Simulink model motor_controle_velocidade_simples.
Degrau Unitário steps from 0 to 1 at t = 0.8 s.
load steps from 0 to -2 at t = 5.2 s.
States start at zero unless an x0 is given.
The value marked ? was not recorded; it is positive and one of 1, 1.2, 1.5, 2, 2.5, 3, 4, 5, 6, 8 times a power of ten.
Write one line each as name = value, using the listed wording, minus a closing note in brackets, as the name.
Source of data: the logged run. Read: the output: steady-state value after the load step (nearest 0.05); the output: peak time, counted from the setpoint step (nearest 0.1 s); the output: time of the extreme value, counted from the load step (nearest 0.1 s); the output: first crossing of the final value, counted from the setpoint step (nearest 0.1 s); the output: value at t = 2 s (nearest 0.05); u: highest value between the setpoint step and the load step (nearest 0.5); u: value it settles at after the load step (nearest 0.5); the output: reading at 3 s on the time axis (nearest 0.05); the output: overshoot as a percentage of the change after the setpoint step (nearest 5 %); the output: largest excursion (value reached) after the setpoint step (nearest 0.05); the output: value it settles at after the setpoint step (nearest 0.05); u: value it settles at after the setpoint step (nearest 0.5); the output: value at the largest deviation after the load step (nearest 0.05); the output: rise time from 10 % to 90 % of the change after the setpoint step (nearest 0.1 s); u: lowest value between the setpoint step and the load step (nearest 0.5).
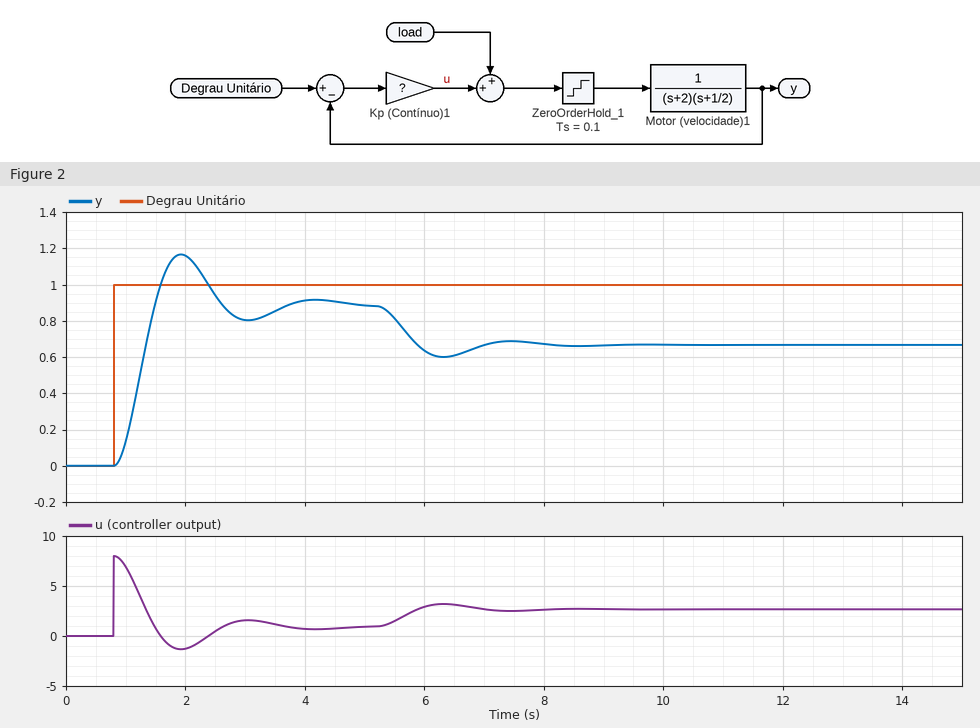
the output: steady-state value after the load step = 0.65
the output: peak time, counted from the setpoint step = 1.1 s
the output: time of the extreme value, counted from the load step = 1.1 s
the output: first crossing of the final value, counted from the setpoint step = 0.7 s
the output: value at t = 2 s = 1.15
u: highest value between the setpoint step and the load step = 8.0
u: value it settles at after the load step = 2.5
the output: reading at 3 s on the time axis = 0.80
the output: overshoot as a percentage of the change after the setpoint step = 30 %
the output: largest excursion (value reached) after the setpoint step = 1.15
the output: value it settles at after the setpoint step = 0.90
u: value it settles at after the setpoint step = 1.0
the output: value at the largest deviation after the load step = 0.60
the output: rise time from 10 % to 90 % of the change after the setpoint step = 0.5 s
u: lowest value between the setpoint step and the load step = -1.5
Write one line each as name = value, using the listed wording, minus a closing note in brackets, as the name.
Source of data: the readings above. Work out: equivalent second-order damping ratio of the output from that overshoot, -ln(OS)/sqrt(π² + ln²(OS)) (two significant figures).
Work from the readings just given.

equivalent second-order damping ratio of the output from that overshoot, -ln(OS)/sqrt(π² + ln²(OS)) = 0.36
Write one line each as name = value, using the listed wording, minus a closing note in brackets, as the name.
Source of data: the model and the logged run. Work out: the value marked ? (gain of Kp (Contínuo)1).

the value marked ? (gain of Kp (Contínuo)1) = 8
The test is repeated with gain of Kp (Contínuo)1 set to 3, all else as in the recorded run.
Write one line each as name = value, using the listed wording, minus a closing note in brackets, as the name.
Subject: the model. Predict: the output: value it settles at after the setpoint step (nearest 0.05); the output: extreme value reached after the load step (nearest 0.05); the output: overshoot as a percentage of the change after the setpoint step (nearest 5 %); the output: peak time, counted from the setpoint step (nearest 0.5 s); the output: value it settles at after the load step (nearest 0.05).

the output: value it settles at after the setpoint step = 0.75
the output: extreme value reached after the load step = 0.20
the output: overshoot as a percentage of the change after the setpoint step = 10 %
the output: peak time, counted from the setpoint step = 2.0 s
the output: value it settles at after the load step = 0.25
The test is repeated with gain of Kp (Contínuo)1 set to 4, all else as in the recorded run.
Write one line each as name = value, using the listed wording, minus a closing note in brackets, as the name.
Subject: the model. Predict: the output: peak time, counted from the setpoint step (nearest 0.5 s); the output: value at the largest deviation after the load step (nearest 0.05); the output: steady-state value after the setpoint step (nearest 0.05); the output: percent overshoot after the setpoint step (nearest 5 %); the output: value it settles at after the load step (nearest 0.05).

the output: peak time, counted from the setpoint step = 1.5 s
the output: value at the largest deviation after the load step = 0.35
the output: steady-state value after the setpoint step = 0.80
the output: percent overshoot after the setpoint step = 15 %
the output: value it settles at after the load step = 0.40
